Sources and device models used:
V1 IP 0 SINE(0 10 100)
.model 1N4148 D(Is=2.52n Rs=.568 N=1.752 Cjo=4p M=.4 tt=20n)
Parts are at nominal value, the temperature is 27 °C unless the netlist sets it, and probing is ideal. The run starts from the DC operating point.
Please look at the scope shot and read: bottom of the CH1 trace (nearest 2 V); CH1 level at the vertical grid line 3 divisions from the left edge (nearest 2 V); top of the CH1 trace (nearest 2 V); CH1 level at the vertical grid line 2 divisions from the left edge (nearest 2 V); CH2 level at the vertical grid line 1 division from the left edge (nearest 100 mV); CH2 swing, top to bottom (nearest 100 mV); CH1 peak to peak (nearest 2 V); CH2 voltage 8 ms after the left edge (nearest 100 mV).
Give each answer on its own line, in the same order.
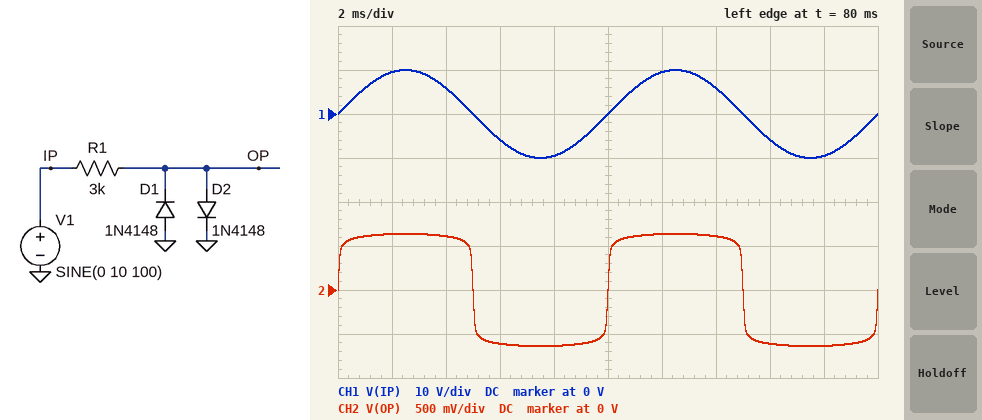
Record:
-10 V
-6 V
10 V
6 V
600 mV
1.3 V
20 V
-600 mV
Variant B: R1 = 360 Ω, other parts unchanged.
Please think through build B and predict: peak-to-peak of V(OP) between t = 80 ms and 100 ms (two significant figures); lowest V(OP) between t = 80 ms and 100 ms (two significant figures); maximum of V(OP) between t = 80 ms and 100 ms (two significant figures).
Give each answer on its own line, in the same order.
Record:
1.5 V
-750 mV
750 mV
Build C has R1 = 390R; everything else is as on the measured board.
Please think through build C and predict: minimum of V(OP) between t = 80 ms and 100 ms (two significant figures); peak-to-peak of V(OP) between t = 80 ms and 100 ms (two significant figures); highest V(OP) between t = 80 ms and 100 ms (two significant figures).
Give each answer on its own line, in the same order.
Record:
-740 mV
1.5 V
740 mV
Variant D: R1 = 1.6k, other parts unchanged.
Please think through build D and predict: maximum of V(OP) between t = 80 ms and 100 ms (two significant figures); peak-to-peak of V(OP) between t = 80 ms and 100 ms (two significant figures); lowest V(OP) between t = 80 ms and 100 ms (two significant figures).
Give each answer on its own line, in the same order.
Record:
670 mV
1.3 V
-670 mV
